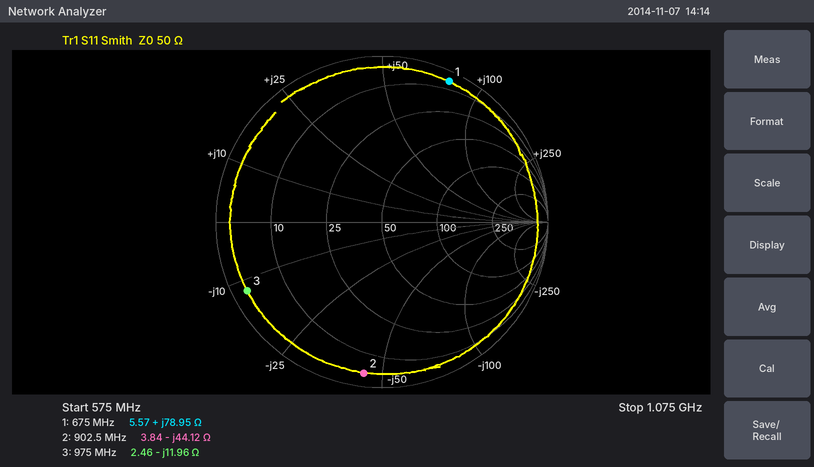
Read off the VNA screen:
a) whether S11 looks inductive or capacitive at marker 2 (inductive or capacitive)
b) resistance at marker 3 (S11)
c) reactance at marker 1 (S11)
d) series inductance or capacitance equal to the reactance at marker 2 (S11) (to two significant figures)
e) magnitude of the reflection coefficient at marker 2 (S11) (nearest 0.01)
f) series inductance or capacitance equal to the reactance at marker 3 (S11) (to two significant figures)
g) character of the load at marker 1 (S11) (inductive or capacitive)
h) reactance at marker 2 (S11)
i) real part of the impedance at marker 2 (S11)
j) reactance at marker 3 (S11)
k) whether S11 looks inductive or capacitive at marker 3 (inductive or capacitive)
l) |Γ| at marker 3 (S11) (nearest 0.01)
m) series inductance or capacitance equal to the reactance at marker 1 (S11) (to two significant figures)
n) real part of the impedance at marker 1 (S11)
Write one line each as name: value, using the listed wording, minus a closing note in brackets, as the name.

whether S11 looks inductive or capacitive at marker 2: capacitive
resistance at marker 3: 2.46 Ω
reactance at marker 1: +78.95 Ω
series inductance or capacitance equal to the reactance at marker 2 (S11): 4.0 pF
magnitude of the reflection coefficient at marker 2 (S11): 0.92
series inductance or capacitance equal to the reactance at marker 3 (S11): 14 pF
character of the load at marker 1 (S11): inductive
reactance at marker 2: -44.12 Ω
real part of the impedance at marker 2: 3.84 Ω
reactance at marker 3: -11.96 Ω
whether S11 looks inductive or capacitive at marker 3: capacitive
|Γ| at marker 3 (S11): 0.91
series inductance or capacitance equal to the reactance at marker 1 (S11): 19 nH
real part of the impedance at marker 1: 5.57 Ω
